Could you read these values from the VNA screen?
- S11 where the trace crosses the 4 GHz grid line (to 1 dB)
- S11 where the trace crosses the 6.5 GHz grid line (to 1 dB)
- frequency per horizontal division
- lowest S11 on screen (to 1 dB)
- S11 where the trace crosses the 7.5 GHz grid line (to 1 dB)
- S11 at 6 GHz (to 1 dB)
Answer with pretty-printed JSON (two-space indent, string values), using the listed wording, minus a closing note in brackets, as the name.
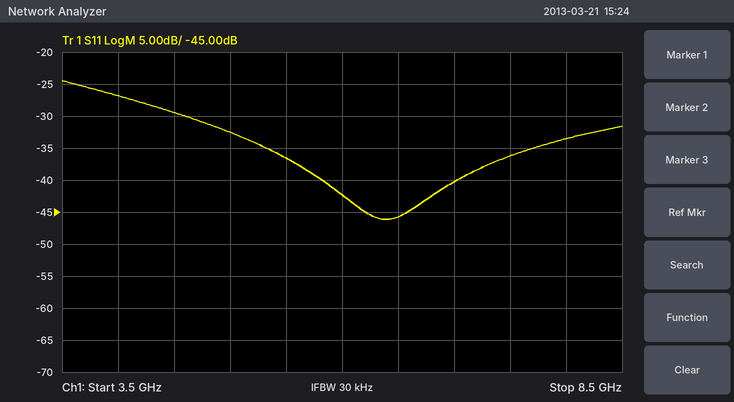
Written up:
{
  "S11 where the trace crosses the 4 GHz grid line": "-27 dB",
  "S11 where the trace crosses the 6.5 GHz grid line": "-46 dB",
  "frequency per horizontal division": "500 MHz",
  "lowest S11 on screen": "-46 dB",
  "S11 where the trace crosses the 7.5 GHz grid line": "-36 dB",
  "S11 at 6 GHz": "-42 dB"
}
